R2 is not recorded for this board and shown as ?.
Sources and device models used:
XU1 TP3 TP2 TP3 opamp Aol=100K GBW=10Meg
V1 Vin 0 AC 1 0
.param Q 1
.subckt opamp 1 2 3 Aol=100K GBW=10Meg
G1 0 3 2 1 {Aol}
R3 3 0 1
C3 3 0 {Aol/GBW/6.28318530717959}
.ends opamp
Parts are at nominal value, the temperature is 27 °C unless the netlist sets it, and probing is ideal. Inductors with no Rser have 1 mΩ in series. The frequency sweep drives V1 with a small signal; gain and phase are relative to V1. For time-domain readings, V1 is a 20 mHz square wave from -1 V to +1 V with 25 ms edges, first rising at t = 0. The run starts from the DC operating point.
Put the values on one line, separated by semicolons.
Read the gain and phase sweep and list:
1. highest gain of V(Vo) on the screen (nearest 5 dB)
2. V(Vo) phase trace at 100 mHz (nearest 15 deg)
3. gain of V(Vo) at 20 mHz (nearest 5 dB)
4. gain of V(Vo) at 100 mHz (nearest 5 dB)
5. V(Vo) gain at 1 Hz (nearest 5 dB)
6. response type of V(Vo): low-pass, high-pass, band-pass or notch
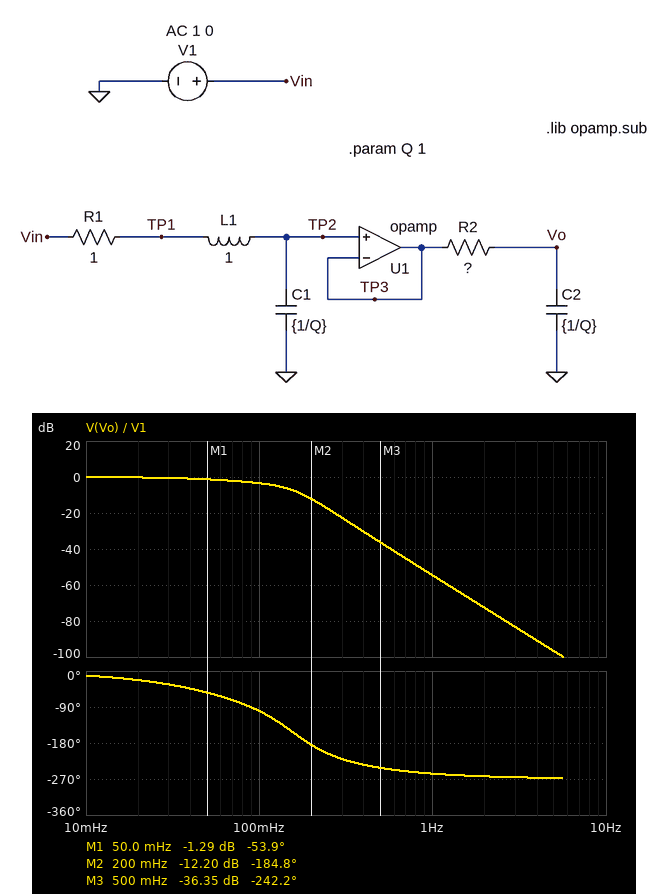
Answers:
0 dB; -105 deg; 0 dB; -5 dB; -55 dB; low-pass
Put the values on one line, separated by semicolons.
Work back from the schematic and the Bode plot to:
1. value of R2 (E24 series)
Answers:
2.2 Ω
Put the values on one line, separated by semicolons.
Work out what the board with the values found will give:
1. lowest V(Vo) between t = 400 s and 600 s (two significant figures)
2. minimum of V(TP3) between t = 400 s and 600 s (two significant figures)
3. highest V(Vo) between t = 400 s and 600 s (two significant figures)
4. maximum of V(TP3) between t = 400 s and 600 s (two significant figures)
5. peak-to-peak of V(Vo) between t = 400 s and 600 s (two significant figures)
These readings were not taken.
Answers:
-1.0 V; -1.3 V; 1.0 V; 1.3 V; 2.0 V
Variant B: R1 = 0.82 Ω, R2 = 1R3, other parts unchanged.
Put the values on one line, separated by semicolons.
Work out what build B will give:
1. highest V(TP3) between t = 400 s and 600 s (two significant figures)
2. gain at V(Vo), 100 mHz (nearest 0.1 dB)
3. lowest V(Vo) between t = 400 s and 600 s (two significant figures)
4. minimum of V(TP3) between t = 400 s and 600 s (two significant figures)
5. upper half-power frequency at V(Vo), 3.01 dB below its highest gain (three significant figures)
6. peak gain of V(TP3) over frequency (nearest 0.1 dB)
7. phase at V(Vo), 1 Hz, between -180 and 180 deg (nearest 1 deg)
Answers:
1.5 V; -0.2 dB; -1.2 V; -1.5 V; 164 mHz; 2.5 dB; 105 deg
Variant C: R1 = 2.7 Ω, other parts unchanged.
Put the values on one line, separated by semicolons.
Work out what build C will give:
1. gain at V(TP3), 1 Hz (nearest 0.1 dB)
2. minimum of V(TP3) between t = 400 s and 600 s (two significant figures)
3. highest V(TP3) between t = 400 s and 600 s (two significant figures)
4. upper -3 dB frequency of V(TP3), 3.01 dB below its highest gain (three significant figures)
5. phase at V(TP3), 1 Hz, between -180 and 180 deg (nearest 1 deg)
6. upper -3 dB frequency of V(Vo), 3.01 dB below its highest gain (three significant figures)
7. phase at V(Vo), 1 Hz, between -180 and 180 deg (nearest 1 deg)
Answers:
-32.5 dB; -1.0 V; 1.0 V; 68.0 mHz; -156 deg; 45.3 mHz; 118 deg
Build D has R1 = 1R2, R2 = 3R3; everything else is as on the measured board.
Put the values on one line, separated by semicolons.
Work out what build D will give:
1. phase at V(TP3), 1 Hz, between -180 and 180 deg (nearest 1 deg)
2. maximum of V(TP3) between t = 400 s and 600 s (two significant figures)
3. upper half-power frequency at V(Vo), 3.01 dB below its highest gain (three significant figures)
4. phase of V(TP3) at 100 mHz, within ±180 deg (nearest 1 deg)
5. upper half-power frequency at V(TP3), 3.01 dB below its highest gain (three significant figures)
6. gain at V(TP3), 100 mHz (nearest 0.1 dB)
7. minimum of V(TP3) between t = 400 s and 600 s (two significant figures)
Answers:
-169 deg; 1.2 V; 50.5 mHz; -51 deg; 177 mHz; 0.3 dB; -1.2 V
